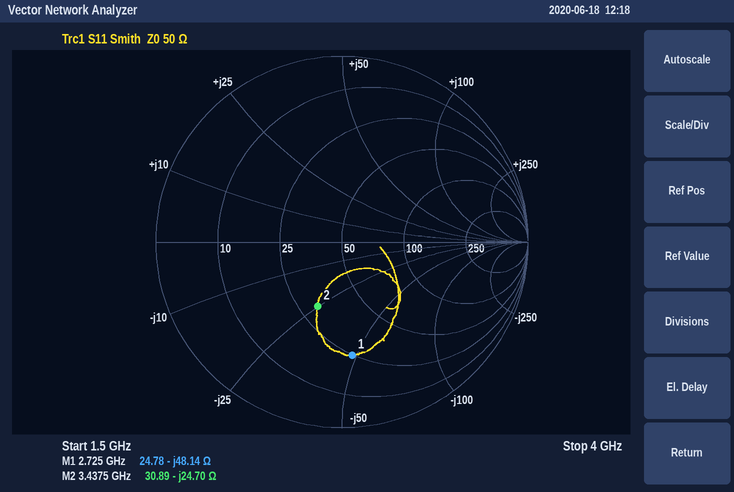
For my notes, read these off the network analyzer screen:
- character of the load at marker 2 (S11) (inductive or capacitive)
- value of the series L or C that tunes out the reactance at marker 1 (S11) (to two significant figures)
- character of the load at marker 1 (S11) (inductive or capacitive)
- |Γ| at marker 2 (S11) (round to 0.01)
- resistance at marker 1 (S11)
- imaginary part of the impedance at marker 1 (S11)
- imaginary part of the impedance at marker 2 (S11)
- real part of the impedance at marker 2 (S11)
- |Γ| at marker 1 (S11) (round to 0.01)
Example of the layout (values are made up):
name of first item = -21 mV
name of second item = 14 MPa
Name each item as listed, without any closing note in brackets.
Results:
character of the load at marker 2 (S11) = capacitive
value of the series L or C that tunes out the reactance at marker 1 (S11) = 2.8 nH
character of the load at marker 1 (S11) = capacitive
|Γ| at marker 2 (S11) = 0.37
resistance at marker 1 = 24.78 Ω
imaginary part of the impedance at marker 1 = -48.14 Ω
imaginary part of the impedance at marker 2 = -24.70 Ω
real part of the impedance at marker 2 = 30.89 Ω
|Γ| at marker 1 (S11) = 0.61
